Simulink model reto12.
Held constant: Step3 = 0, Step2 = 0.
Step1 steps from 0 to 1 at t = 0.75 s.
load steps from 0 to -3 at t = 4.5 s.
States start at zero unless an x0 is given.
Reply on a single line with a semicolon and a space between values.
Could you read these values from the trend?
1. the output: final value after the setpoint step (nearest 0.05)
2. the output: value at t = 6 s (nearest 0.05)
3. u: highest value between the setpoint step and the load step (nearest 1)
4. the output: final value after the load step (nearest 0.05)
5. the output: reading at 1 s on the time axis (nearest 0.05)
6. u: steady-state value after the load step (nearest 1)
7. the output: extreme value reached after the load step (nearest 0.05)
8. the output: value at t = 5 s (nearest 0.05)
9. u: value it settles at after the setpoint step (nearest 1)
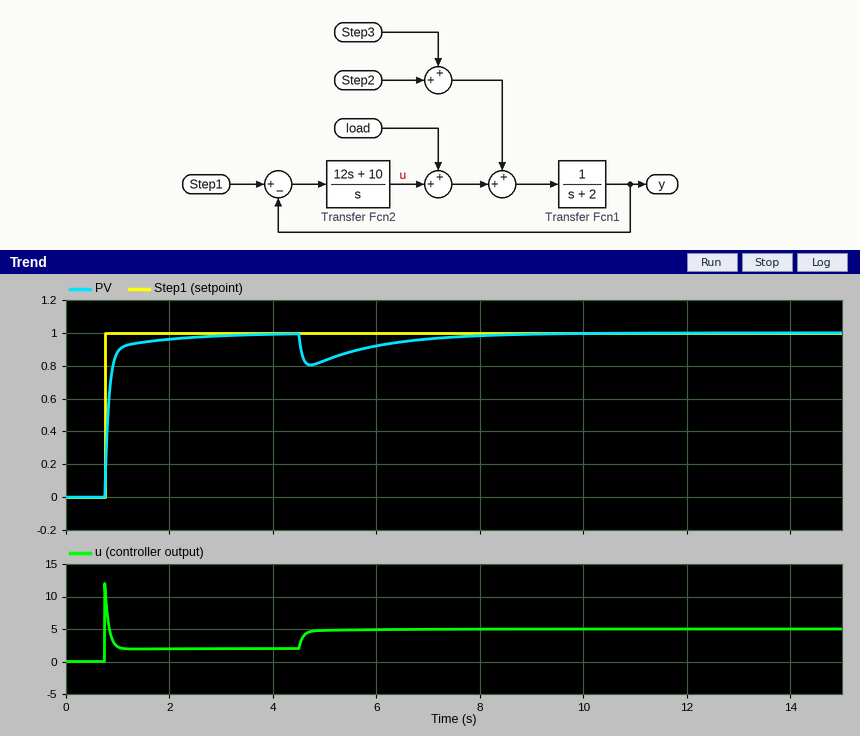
1.00; 0.90; 12; 1.00; 0.90; 5; 0.80; 0.85; 2
